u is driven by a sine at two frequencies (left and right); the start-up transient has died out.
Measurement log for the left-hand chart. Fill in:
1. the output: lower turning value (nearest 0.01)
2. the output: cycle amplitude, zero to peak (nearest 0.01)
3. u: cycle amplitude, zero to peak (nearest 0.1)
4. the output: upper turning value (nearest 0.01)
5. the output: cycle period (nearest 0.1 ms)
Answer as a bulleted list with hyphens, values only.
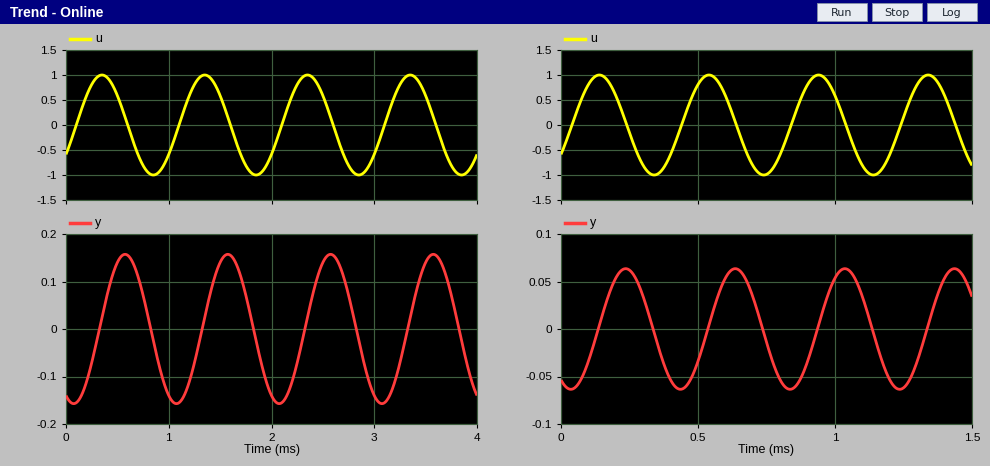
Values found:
- -0.16
- 0.16
- 1.0
- 0.16
- 1.0 ms
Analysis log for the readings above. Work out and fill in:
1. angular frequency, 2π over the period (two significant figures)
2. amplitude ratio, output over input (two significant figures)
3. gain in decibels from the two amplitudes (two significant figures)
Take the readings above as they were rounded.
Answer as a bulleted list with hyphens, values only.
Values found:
- 6.3 rad/ms
- 0.16
- -16 dB
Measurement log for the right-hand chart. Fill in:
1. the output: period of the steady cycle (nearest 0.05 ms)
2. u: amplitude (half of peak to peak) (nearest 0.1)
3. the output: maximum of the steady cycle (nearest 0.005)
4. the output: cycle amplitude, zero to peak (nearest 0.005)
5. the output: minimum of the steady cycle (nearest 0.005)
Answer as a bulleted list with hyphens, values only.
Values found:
- 0.40 ms
- 1.0
- 0.065
- 0.065
- -0.065
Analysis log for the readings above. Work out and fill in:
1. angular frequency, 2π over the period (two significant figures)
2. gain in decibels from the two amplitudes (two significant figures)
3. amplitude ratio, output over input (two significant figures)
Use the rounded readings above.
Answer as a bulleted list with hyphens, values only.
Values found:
- 16 rad/ms
- -24 dB
- 0.065
